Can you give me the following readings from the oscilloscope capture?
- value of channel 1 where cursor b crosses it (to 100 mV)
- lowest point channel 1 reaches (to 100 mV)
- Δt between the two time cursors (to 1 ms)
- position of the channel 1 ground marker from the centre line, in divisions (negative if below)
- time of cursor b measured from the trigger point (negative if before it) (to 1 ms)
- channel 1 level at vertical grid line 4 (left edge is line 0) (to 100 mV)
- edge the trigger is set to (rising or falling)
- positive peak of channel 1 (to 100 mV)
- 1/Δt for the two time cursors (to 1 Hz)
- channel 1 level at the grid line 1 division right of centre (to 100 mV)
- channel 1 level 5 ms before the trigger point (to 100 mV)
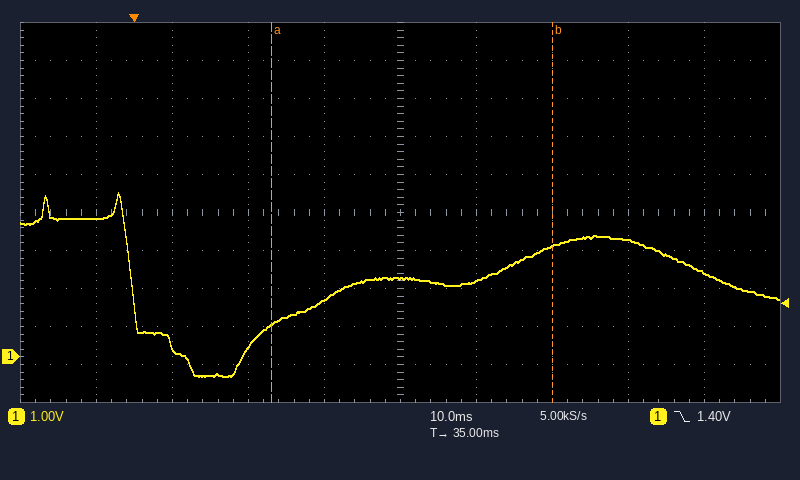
2.9 V
-500 mV
37 ms
-3.8 div
+55 ms
1.5 V
falling
4.3 V
27 Hz
2.0 V
3.6 V
